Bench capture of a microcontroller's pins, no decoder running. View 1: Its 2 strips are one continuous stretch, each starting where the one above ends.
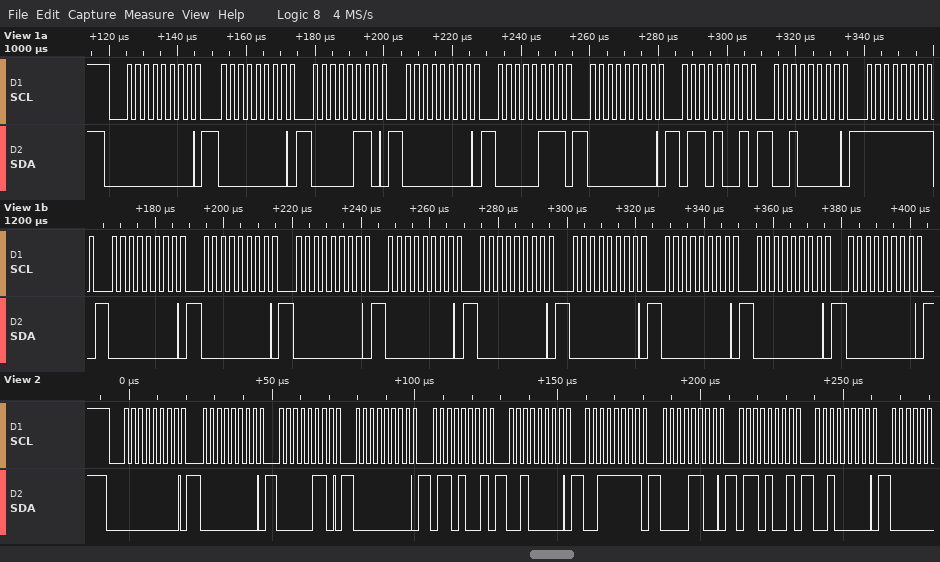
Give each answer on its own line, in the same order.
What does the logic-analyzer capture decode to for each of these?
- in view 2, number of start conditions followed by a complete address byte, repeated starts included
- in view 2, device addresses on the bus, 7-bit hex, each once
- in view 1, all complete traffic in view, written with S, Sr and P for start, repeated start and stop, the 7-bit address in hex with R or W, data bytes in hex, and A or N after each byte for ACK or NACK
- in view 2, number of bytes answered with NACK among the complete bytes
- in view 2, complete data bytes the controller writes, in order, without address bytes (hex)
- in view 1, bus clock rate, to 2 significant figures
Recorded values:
1
0x00
S 00W A 00 A 06 A 00 A 07 A 00 A 69 A 20 A FF A 00 A 00 A 00 A 00 A 00 A 00 A 00 A 00 A 00 A
0
00 06 00 69 20 3F 0C 69 20
400 kHz
